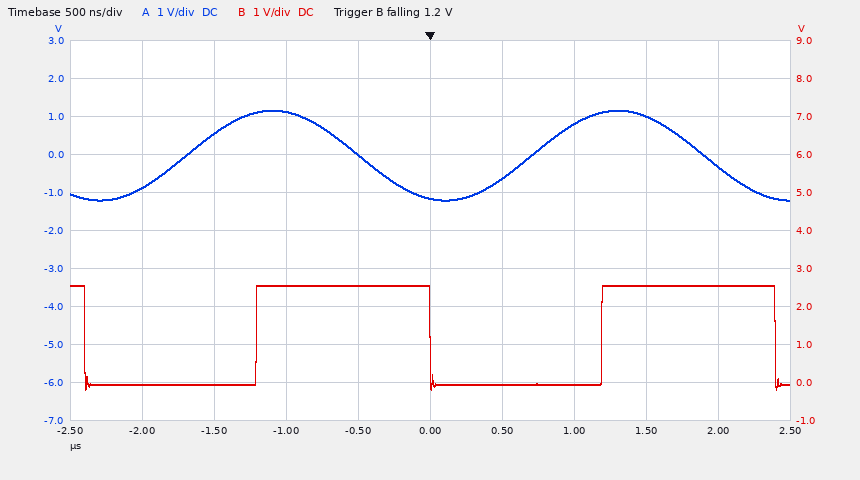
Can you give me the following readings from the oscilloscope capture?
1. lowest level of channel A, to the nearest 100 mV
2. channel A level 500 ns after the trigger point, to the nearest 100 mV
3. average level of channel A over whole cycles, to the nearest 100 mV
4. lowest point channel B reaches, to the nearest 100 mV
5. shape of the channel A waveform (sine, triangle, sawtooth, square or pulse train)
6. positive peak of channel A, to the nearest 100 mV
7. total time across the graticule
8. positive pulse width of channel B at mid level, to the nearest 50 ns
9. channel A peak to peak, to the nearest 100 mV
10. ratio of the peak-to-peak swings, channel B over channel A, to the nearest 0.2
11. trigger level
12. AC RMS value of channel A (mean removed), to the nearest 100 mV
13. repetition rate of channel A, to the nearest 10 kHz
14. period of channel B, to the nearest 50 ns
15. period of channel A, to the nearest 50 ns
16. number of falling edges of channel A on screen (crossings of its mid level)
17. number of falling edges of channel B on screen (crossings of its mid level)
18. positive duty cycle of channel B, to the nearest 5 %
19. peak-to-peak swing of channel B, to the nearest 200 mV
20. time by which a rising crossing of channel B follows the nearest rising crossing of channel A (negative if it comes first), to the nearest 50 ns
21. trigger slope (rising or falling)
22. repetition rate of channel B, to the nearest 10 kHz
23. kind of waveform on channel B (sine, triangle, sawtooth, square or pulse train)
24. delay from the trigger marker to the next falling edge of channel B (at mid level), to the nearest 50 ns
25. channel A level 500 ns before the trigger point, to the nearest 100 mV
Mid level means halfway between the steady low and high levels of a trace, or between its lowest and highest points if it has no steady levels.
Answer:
-1.2 V
-600 mV
0.0 V
-200 mV
sine
1.2 V
5 µs
1.20 µs
2.4 V
1.2
1.2 V
800 mV
420 kHz
2.40 µs
2.40 µs
2
3
50 %
2.8 V
+500 ns
falling
420 kHz
square
2.40 µs
0.0 V
